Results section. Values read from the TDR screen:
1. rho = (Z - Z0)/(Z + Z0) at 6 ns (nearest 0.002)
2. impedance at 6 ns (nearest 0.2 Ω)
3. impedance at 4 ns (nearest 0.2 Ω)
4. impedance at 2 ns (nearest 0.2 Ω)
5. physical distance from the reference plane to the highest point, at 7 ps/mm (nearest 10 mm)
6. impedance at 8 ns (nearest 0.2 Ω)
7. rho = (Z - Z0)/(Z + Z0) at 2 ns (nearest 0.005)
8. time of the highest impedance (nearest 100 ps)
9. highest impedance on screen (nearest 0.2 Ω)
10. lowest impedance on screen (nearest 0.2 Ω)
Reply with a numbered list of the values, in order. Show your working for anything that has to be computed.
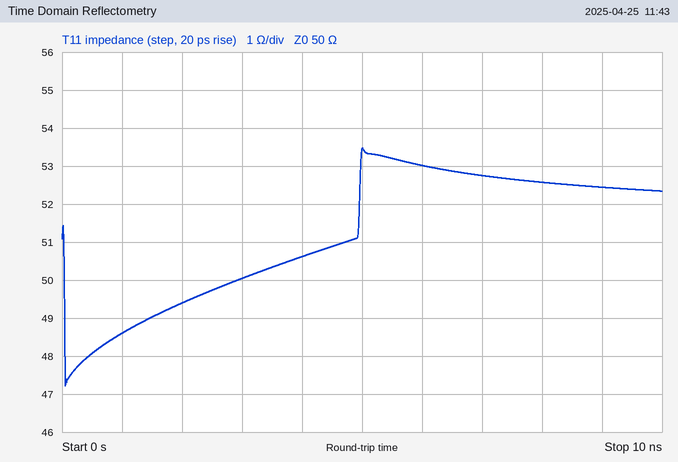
1. (53 − 50)/(53 + 50) ≈ +0.0291, so +0.030 to the nearest 0.002
2. 53.0 Ω
3. 50.6 Ω
4. 49.4 Ω
5. 5.0 ns / 2 / 7 ps/mm ≈ 357 mm, so 360 mm to the nearest 10 mm
6. 52.6 Ω
7. (49.4 − 50)/(49.4 + 50) ≈ -0.00604, so -0.005 to the nearest 0.005
8. 5.0 ns
9. 53.4 Ω
10. 47.2 Ω
